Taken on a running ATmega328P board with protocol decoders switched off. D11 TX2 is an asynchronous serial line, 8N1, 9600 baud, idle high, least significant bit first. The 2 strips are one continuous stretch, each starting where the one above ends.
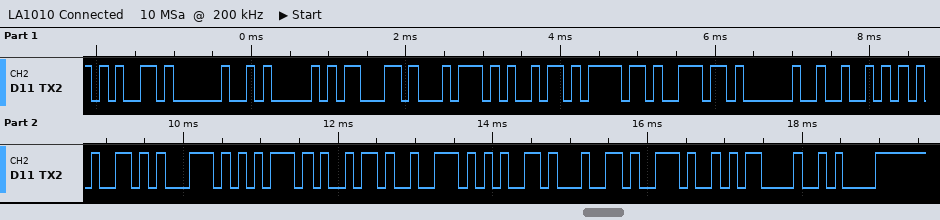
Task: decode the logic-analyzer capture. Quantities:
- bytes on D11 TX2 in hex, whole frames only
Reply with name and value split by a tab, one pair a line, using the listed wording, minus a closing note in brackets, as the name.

bytes on D11 TX2 in hex, whole frames only	65 20 41 63 74 69 6F 6E 20 52 65 71 75 69 72 65 64 2E 0D 0A
